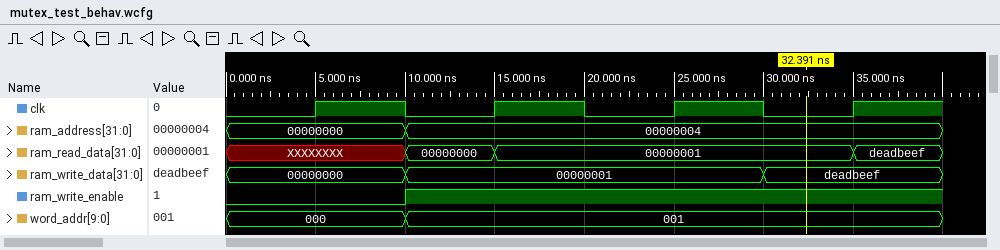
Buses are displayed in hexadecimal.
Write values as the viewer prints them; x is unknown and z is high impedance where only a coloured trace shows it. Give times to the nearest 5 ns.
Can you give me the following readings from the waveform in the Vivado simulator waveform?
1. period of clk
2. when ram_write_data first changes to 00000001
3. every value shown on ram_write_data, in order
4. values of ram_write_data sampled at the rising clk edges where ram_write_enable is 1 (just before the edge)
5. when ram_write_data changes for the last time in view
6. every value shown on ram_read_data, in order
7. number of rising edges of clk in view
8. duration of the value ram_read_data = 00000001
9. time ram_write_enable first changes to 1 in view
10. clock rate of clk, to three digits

10 ns
10 ns
00000000, 00000001, deadbeef
00000001, 00000001, deadbeef
30 ns
XXXXXXXX, 00000000, 00000001, deadbeef
4
20 ns
10 ns
100 MHz
